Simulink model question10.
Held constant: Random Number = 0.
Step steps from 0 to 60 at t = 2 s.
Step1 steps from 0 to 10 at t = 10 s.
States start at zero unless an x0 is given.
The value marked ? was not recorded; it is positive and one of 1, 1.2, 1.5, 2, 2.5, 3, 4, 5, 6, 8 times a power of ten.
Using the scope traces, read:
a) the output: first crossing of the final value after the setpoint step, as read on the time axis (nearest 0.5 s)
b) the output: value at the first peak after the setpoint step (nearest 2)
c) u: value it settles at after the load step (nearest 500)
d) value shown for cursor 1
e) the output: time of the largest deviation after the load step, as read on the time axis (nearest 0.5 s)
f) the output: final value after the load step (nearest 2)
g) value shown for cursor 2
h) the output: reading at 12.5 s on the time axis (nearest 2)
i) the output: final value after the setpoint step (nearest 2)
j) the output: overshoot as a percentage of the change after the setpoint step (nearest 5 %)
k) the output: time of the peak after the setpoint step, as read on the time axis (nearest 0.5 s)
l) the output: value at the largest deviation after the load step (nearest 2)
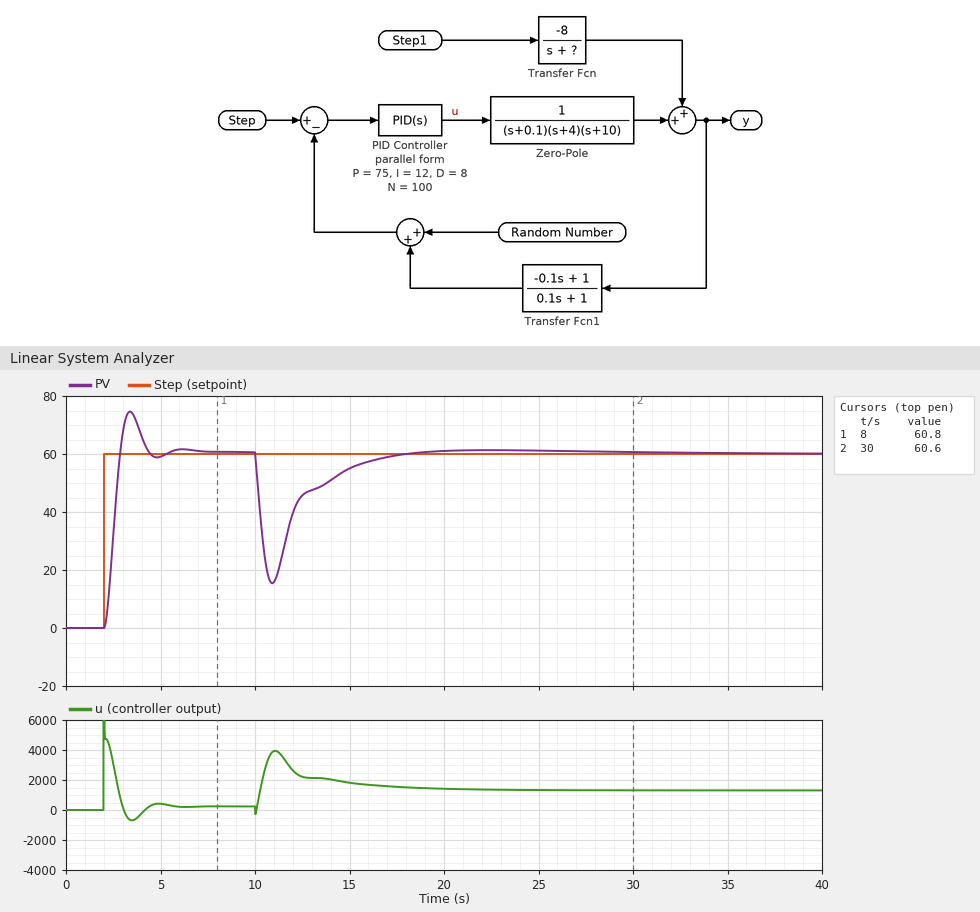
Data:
3.0 s
74
1500
60.8
11.0 s
60
60.6
46
60
25 %
3.5 s
16
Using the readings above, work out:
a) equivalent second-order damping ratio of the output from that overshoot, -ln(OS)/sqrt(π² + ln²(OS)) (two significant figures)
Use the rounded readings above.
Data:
0.40
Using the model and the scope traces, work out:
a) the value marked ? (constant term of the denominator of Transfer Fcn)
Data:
0.3
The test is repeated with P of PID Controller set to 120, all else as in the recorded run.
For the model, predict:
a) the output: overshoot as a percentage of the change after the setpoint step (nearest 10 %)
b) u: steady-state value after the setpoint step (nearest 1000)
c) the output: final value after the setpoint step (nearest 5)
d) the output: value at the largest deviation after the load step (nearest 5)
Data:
50 %
0
60
20
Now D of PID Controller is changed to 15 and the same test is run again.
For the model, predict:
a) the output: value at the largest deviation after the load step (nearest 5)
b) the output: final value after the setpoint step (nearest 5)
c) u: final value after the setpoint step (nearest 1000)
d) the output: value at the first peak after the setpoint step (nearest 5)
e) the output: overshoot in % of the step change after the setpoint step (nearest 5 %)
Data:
20
60
0
70
15 %
